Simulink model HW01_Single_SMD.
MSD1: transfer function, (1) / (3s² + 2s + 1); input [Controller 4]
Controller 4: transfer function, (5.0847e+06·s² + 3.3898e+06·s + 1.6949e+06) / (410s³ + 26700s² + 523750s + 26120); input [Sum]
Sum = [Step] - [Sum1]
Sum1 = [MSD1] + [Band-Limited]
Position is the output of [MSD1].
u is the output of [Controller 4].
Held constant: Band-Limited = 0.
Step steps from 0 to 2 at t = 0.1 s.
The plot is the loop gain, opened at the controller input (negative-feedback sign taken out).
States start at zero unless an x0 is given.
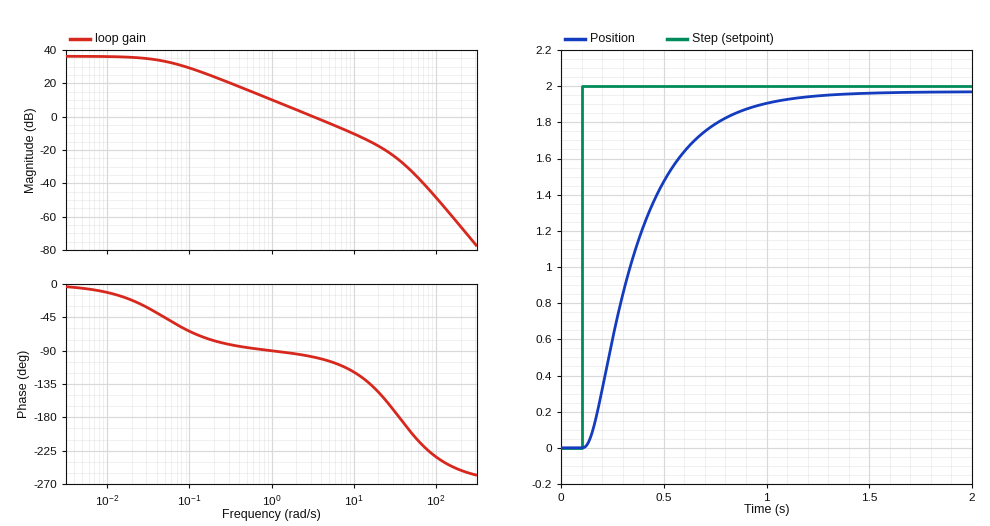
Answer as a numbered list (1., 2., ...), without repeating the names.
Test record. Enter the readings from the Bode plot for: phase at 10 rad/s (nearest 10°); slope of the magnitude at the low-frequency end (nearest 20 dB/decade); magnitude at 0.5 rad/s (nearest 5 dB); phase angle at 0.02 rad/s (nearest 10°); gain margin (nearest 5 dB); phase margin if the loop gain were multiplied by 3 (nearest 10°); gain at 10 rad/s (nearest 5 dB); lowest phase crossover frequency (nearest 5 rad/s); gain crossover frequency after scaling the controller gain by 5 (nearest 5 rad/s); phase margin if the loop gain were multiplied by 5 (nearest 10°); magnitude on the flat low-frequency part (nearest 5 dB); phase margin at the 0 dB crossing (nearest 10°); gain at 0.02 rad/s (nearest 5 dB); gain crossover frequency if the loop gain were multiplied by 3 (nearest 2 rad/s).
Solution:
1. -120°
2. 0 dB/decade
3. 15 dB
4. -20°
5. 25 dB
6. 60°
7. -10 dB
8. 35 rad/s
9. 15 rad/s
10. 50°
11. 35 dB
12. 80°
13. 35 dB
14. 10 rad/s
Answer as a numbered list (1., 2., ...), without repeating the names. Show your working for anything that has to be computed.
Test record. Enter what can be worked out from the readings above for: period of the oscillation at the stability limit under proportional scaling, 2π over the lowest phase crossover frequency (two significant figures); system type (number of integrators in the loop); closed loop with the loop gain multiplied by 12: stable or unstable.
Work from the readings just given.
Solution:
1. 2π / 35 = 0.18 s
2. 0
3. stable
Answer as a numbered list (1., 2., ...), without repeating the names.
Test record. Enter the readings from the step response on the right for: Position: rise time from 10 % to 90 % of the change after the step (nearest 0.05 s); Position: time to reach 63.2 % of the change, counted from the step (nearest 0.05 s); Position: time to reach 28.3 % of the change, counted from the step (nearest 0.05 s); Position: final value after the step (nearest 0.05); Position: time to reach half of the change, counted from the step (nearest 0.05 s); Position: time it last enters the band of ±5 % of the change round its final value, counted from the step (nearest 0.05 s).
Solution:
1. 0.55 s
2. 0.30 s
3. 0.15 s
4. 1.95
5. 0.25 s
6. 0.80 s
